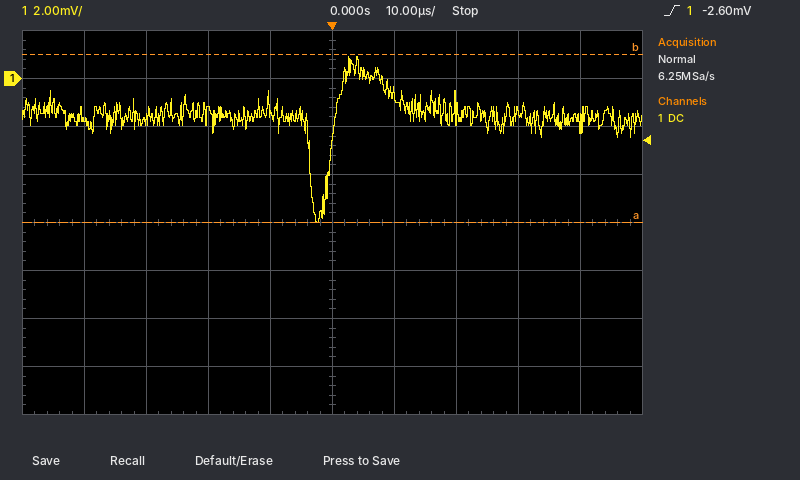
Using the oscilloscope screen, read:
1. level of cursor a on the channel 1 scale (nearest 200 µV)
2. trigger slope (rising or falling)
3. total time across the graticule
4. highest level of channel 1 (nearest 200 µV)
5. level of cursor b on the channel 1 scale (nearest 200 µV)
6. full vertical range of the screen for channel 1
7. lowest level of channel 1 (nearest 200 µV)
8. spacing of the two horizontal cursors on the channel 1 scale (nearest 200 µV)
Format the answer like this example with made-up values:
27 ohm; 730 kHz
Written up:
-6.0 mV; rising; 100 µs; 1.0 mV; 1.0 mV; 16 mV; -6.0 mV; 7.0 mV
